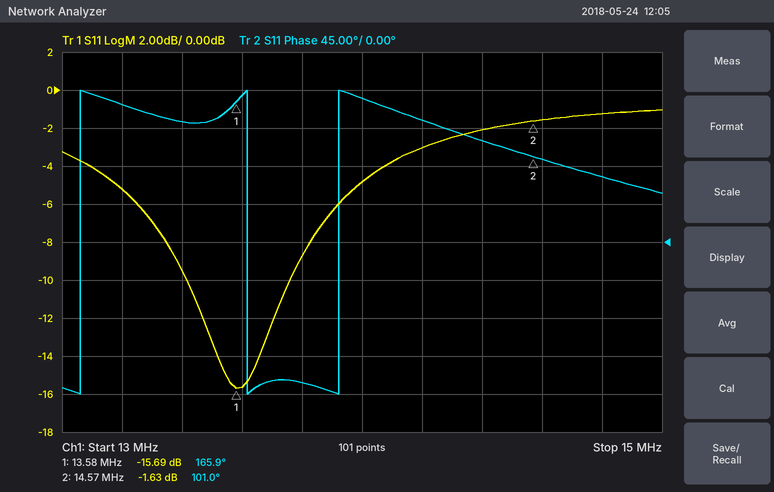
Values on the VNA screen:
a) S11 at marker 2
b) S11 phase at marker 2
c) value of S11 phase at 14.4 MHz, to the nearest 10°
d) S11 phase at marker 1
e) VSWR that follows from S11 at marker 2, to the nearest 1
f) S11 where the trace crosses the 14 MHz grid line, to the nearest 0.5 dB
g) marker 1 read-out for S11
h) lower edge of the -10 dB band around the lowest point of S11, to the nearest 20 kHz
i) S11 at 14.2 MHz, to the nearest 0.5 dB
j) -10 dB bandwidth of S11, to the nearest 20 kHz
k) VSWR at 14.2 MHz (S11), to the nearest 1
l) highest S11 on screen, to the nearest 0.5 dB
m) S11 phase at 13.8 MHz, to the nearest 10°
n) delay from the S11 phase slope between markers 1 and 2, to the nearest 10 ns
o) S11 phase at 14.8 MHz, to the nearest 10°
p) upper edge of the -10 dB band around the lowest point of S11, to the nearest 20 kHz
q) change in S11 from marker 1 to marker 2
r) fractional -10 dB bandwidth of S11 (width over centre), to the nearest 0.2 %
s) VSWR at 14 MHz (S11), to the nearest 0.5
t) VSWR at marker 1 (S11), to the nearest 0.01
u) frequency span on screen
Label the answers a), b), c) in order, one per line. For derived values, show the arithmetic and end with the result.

a) -1.63 dB
b) 101.0°
c) 120°
d) 165.9°
e) (1 + 0.8289)/(1 − 0.8289) ≈ 11
f) -5.0 dB
g) -15.69 dB
h) 13.42 MHz
i) -3.0 dB
j) 13.76 MHz − 13.42 MHz = 340 kHz
k) |Γ| = 10^(-3/20) = 0.7079; VSWR = (1 + 0.7079)/(1 − 0.7079) ≈ 6
l) -1.0 dB
m) -170°
n) −(101° − (165.9°))/(360° × 990 kHz) ≈ 182 ns, so 180 ns to the nearest 10 ns
o) 80°
p) 13.76 MHz
q) -1.63 − (-15.69) = 14.06 dB
r) 340 kHz / 13.59 MHz ≈ 2.50 %, so 2.6 % to the nearest 0.2 %
s) |Γ| = 10^(-5/20) = 0.5623; VSWR = (1 + 0.5623)/(1 − 0.5623) ≈ 3.57, so 3.5 to the nearest 0.5
t) (1 + 0.1642)/(1 − 0.1642) ≈ 1.39
u) 2 MHz
